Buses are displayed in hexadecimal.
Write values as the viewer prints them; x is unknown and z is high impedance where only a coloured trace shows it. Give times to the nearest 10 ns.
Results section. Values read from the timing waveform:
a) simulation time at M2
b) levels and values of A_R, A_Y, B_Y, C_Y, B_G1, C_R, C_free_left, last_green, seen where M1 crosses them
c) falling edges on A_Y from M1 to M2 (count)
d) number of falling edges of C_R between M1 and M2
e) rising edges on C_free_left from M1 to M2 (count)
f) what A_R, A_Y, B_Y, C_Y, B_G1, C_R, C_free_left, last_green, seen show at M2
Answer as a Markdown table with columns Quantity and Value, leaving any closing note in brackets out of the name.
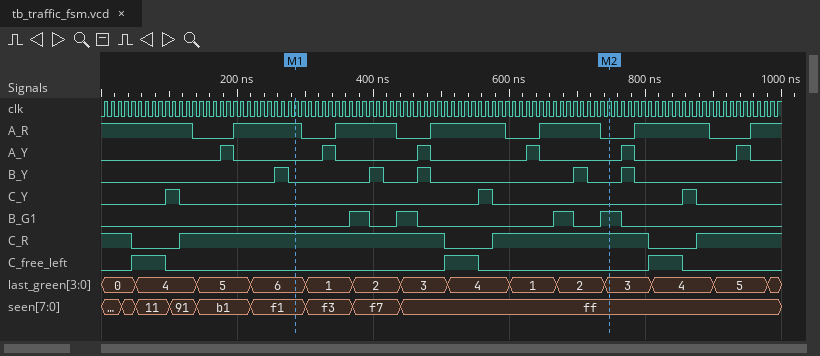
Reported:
| Quantity | Value |
|---|---|
| simulation time at M2 | 750 ns |
| levels and values of A_R, A_Y, B_Y, C_Y, B_G1, C_R, C_free_left, last_green, seen where M1 crosses them | A_R=1, A_Y=0, B_Y=0, C_Y=0, B_G1=0, C_R=1, C_free_left=0, last_green=6, seen=f1 |
| falling edges on A_Y from M1 to M2 | 3 |
| number of falling edges of C_R between M1 and M2 | 1 |
| rising edges on C_free_left from M1 to M2 | 1 |
| what A_R, A_Y, B_Y, C_Y, B_G1, C_R, C_free_left, last_green, seen show at M2 | A_R=0, A_Y=0, B_Y=0, C_Y=0, B_G1=1, C_R=1, C_free_left=0, last_green=3, seen=ff |
